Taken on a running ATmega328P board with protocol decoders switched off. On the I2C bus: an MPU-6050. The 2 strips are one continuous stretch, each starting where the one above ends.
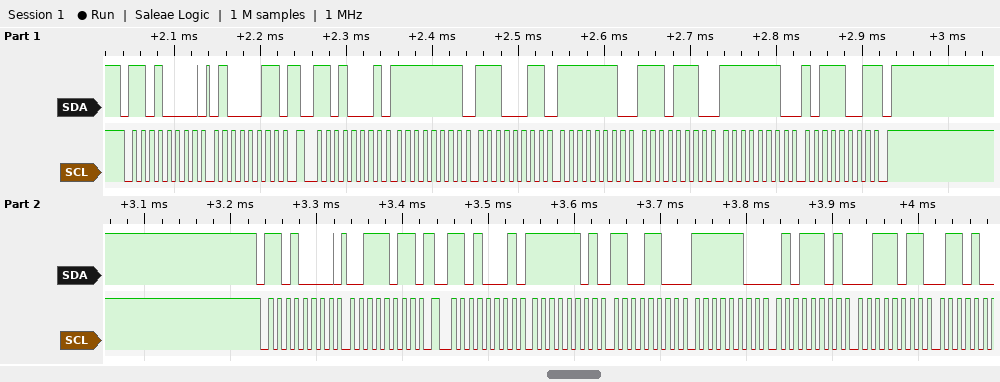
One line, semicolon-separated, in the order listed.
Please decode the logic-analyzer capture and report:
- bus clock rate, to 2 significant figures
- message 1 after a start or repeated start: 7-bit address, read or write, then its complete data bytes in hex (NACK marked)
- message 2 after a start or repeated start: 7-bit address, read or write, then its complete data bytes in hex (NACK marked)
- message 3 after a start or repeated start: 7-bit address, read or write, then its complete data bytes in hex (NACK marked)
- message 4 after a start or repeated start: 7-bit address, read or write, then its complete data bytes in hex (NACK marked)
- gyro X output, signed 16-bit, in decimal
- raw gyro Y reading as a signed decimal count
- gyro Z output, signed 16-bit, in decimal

100 kHz; 0x68 write: 43; 0x68 read: FF E3 FE EE FE B9 NACK; 0x68 write: 3B; 0x68 read: FD CC FC 5D 3B; -29; -274; -327
